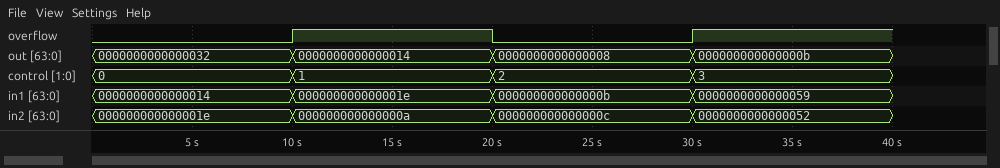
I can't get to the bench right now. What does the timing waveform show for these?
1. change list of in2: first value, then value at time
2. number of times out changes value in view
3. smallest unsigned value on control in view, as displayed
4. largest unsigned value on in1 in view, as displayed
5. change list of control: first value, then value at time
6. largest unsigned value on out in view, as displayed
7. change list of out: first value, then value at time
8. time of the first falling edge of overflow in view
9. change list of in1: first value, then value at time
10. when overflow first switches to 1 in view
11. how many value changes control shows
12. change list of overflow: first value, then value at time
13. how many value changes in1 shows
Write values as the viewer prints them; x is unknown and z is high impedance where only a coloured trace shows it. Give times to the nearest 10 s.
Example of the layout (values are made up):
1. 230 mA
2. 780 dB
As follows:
1. 000000000000001e, 000000000000000a at 10 s, 000000000000000c at 20 s, 0000000000000052 at 30 s
2. 3
3. 0
4. 0000000000000059
5. 0, 1 at 10 s, 2 at 20 s, 3 at 30 s
6. 0000000000000032
7. 0000000000000032, 0000000000000014 at 10 s, 0000000000000008 at 20 s, 000000000000000b at 30 s
8. 20 s
9. 0000000000000014, 000000000000001e at 10 s, 000000000000000b at 20 s, 0000000000000059 at 30 s
10. 10 s
11. 3
12. 0, 1 at 10 s, 0 at 20 s, 1 at 30 s
13. 3
